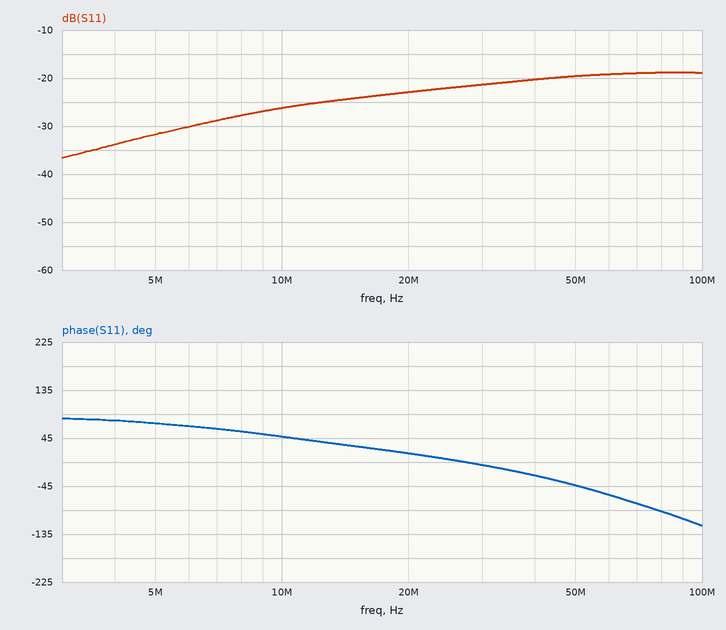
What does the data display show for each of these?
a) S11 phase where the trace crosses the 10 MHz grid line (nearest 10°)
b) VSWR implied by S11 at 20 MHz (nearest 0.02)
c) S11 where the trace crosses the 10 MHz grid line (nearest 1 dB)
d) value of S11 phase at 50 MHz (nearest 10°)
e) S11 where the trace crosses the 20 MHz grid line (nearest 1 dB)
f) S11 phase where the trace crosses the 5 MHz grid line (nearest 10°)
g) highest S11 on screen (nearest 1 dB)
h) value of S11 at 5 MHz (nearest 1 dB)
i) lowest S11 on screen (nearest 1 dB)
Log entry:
50°
1.16
-26 dB
-40°
-23 dB
70°
-19 dB
-32 dB
-37 dB
